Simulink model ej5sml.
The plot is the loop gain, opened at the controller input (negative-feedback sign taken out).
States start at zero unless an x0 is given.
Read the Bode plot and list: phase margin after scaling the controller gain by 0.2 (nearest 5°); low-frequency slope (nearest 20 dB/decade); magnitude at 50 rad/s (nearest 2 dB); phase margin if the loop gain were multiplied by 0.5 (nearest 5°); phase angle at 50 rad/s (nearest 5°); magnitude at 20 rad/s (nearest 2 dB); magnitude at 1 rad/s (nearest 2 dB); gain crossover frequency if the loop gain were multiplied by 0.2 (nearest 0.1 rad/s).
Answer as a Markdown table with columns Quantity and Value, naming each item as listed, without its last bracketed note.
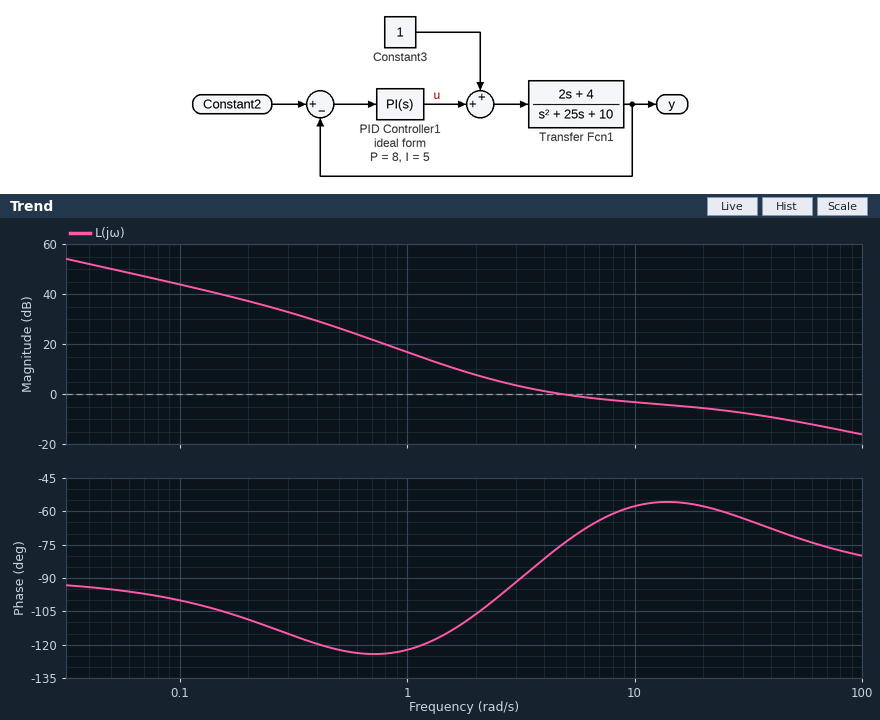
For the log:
| Quantity | Value |
|---|---|
| phase margin after scaling the controller gain by 0.2 | 60° |
| low-frequency slope | -20 dB/decade |
| magnitude at 50 rad/s | -10 dB |
| phase margin if the loop gain were multiplied by 0.5 | 80° |
| phase angle at 50 rad/s | -70° |
| magnitude at 20 rad/s | -6 dB |
| magnitude at 1 rad/s | 16 dB |
| gain crossover frequency if the loop gain were multiplied by 0.2 | 1.2 rad/s |
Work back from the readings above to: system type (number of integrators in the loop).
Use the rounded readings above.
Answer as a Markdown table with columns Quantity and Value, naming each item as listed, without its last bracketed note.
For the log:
| Quantity | Value |
|---|---|
| system type | 1 |
